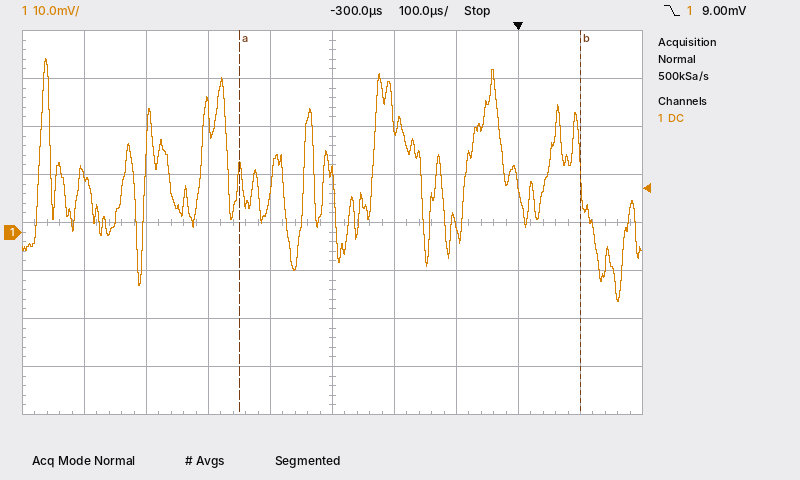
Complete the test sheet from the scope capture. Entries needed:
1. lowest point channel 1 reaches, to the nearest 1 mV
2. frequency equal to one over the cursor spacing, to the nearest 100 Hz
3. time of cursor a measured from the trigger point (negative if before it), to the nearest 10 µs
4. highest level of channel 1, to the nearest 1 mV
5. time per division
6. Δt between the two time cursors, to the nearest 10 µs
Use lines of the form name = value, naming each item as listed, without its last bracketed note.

lowest point channel 1 reaches, to the nearest 1 mV = -14 mV
frequency equal to one over the cursor spacing, to the nearest 100 Hz = 1.8 kHz
time of cursor a measured from the trigger point (negative if before it), to the nearest 10 µs = -450 µs
highest level of channel 1, to the nearest 1 mV = 36 mV
time per division = 100 µs
Δt between the two time cursors, to the nearest 10 µs = 550 µs
